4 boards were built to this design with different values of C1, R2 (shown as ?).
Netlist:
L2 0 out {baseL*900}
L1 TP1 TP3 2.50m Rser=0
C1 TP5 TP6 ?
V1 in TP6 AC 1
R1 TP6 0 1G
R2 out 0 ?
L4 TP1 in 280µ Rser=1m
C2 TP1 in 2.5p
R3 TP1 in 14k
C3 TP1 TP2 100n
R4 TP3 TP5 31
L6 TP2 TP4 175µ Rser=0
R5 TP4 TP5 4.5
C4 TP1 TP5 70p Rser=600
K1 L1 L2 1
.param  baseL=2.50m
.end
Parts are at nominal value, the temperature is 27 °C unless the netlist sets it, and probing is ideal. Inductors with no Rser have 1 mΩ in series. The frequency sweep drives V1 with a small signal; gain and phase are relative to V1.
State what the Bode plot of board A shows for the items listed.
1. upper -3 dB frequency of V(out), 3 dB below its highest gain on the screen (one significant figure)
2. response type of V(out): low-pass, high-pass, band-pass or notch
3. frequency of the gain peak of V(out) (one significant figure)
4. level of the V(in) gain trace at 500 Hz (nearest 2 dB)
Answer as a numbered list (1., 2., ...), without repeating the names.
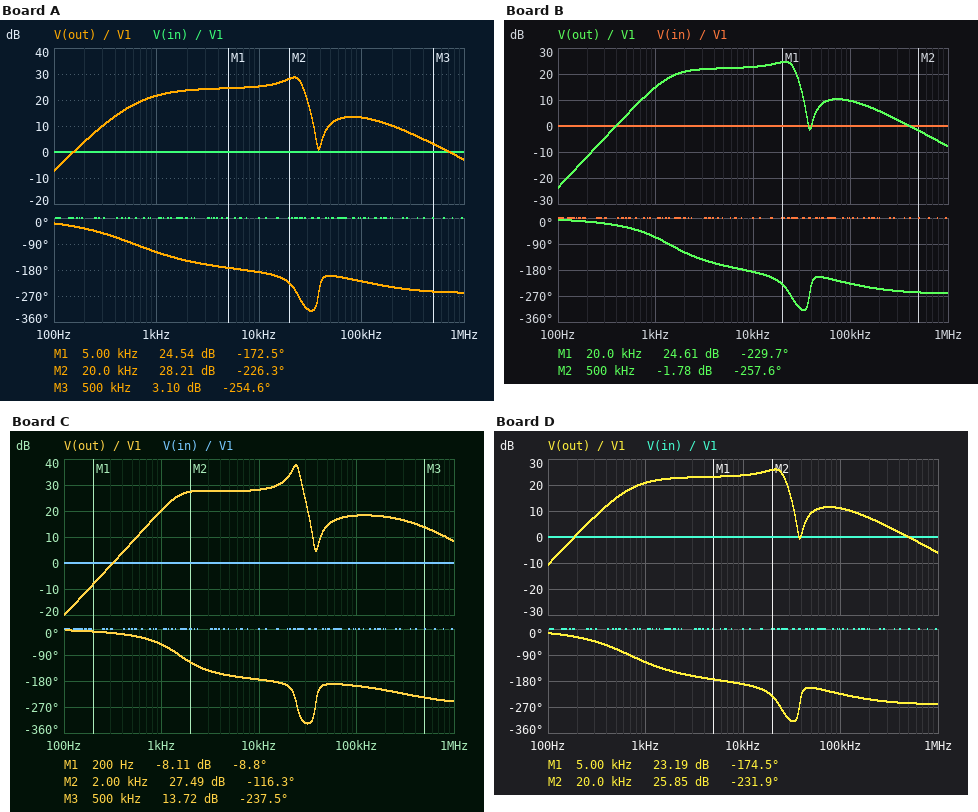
1. 30 kHz
2. band-pass
3. 20 kHz
4. 0 dB
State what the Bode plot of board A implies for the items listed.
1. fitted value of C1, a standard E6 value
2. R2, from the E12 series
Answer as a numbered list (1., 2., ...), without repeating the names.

1. 15 µF
2. 39 kΩ
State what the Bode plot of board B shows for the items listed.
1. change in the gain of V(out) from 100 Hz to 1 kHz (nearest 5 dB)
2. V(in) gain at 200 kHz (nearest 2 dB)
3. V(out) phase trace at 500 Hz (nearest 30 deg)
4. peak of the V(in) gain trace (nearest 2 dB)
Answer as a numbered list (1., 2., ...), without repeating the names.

1. 40 dB
2. 0 dB
3. -30 deg
4. 0 dB
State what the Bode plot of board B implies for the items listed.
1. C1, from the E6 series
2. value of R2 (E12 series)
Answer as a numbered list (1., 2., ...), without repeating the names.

1. 2.2 µF
2. 22 kΩ
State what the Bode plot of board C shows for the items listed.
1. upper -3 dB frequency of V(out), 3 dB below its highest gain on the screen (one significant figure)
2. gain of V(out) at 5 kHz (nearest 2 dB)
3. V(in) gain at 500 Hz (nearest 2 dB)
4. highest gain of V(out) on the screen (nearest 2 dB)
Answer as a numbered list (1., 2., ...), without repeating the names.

1. 30 kHz
2. 28 dB
3. 0 dB
4. 38 dB
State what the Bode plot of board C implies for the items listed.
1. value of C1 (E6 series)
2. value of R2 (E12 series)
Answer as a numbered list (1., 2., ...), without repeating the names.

1. 3.3 µF
2. 150 kΩ
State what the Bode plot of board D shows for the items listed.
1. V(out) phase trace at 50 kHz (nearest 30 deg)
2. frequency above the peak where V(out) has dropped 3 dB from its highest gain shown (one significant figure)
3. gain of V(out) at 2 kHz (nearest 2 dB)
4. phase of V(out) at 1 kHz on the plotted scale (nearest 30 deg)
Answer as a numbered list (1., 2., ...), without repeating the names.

1. -210 deg
2. 30 kHz
3. 22 dB
4. -120 deg
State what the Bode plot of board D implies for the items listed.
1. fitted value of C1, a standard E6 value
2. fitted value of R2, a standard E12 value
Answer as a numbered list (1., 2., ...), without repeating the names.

1. 10 µF
2. 27 kΩ
